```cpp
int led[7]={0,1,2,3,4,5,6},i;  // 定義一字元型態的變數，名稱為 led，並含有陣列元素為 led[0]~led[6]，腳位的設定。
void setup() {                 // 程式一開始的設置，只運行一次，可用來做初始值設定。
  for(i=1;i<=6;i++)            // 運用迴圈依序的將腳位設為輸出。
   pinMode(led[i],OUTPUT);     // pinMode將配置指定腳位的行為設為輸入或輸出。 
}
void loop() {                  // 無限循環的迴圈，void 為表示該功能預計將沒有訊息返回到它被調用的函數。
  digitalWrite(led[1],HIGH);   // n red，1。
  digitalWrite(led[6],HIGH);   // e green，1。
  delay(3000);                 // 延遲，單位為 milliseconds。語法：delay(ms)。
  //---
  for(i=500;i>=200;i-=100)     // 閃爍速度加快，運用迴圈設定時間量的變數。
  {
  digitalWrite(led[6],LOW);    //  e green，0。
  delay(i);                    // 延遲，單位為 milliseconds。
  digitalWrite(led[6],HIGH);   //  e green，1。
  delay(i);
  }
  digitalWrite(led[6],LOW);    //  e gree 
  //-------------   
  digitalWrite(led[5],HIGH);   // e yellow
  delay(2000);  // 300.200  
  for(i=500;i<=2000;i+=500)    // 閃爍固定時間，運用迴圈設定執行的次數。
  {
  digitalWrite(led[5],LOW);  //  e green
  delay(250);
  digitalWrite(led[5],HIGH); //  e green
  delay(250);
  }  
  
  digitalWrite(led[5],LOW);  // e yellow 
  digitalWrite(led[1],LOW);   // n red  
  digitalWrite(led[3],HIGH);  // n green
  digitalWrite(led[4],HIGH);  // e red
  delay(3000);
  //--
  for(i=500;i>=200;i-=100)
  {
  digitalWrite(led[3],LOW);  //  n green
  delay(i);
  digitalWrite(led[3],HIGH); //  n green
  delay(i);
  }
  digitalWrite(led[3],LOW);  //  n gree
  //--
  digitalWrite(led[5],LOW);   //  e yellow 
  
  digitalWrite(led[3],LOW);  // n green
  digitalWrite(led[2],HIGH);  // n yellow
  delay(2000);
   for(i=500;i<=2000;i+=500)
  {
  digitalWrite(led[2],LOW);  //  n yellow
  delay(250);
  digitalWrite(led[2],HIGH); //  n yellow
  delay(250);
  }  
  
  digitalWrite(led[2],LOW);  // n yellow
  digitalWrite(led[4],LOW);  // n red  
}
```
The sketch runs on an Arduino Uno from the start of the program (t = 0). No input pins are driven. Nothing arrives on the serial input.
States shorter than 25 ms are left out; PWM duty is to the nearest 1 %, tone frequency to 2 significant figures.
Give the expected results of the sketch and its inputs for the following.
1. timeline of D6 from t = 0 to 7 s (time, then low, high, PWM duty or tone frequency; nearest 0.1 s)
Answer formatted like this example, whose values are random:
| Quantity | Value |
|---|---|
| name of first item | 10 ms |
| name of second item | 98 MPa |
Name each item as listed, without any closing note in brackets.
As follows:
| Quantity | Value |
|---|---|
| timeline of D6 from t = 0 to 7 s | 0 s high; 3 s low; 3.5 s high; 4 s low; 4.4 s high; 4.8 s low; 5.1 s high; 5.4 s low; 5.6 s high; 5.8 s low |
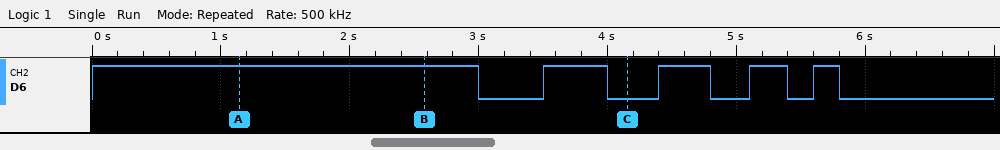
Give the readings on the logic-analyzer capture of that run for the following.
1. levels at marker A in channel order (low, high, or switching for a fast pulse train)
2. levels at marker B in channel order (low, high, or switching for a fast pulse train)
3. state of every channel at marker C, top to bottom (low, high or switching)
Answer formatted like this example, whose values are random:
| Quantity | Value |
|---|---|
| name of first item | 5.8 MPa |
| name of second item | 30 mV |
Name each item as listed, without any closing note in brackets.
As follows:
| Quantity | Value |
|---|---|
| levels at marker A in channel order | D6 high |
| levels at marker B in channel order | D6 high |
| state of every channel at marker C, top to bottom | D6 low |
